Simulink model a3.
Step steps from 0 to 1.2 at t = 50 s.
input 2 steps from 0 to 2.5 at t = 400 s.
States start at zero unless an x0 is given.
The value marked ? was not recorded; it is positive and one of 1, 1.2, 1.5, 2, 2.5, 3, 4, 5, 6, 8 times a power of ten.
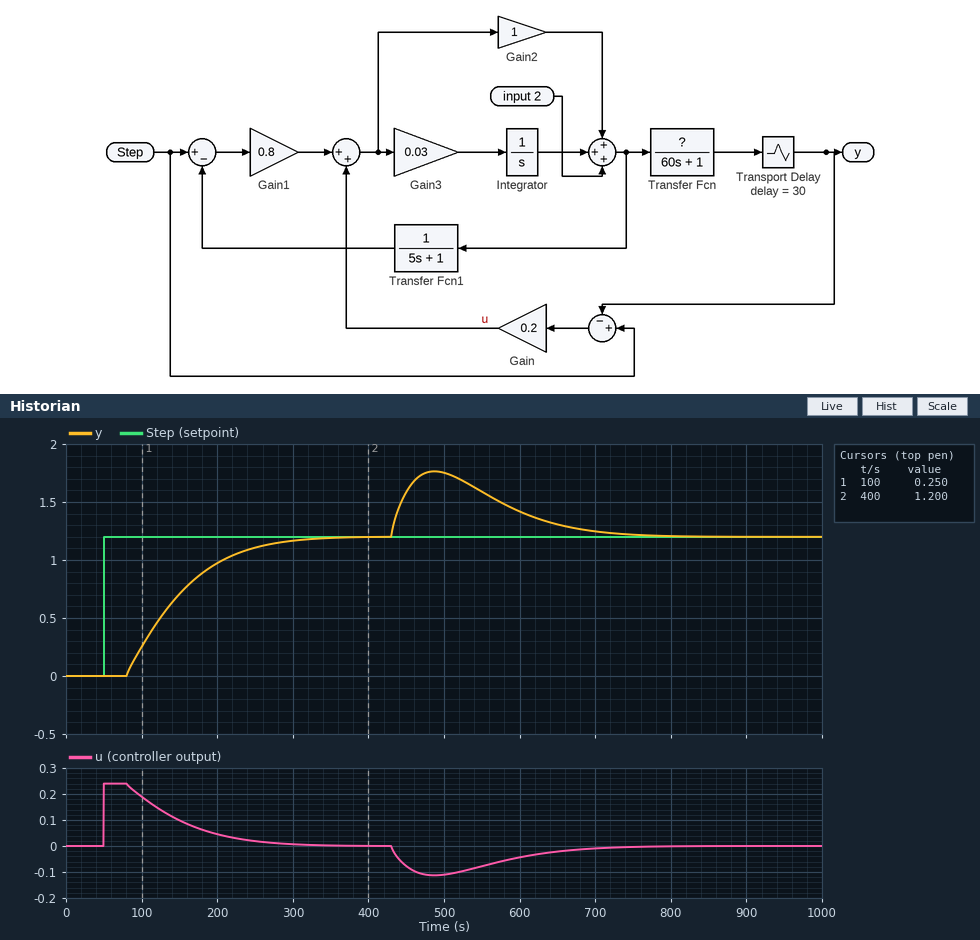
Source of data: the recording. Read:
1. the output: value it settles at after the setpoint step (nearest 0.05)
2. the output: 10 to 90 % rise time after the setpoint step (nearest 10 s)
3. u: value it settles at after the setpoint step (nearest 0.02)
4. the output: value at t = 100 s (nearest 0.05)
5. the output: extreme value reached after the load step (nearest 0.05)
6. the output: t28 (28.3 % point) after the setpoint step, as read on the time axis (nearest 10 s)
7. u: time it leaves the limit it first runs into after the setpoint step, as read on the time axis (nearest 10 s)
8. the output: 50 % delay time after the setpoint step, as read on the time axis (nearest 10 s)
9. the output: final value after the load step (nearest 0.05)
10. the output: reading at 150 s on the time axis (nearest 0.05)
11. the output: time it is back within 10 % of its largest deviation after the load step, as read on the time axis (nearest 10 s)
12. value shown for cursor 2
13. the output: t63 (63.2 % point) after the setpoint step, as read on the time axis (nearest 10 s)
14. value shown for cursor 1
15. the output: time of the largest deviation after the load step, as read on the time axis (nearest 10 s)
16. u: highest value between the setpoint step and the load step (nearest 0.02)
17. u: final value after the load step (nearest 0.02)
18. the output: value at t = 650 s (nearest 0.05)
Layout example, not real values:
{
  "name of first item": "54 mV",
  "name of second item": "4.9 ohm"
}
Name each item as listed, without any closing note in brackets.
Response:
{
  "the output: value it settles at after the setpoint step": "1.20",
  "the output: 10 to 90 % rise time after the setpoint step": "150 s",
  "u: value it settles at after the setpoint step": "0.00",
  "the output: value at t = 100 s": "0.25",
  "the output: extreme value reached after the load step": "1.75",
  "the output: t28 (28.3 % point) after the setpoint step, as read on the time axis": "110 s",
  "u: time it leaves the limit it first runs into after the setpoint step, as read on the time axis": "80 s",
  "the output: 50 % delay time after the setpoint step, as read on the time axis": "140 s",
  "the output: final value after the load step": "1.20",
  "the output: reading at 150 s on the time axis": "0.70",
  "the output: time it is back within 10 % of its largest deviation after the load step, as read on the time axis": "690 s",
  "value shown for cursor 2": "1.200",
  "the output: t63 (63.2 % point) after the setpoint step, as read on the time axis": "160 s",
  "value shown for cursor 1": "0.250",
  "the output: time of the largest deviation after the load step, as read on the time axis": "490 s",
  "u: highest value between the setpoint step and the load step": "0.24",
  "u: final value after the load step": "0.00",
  "the output: value at t = 650 s": "1.30"
}
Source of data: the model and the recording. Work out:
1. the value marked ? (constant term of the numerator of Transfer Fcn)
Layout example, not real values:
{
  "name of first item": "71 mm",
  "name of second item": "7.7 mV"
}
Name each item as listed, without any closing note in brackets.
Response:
{
  "the value marked ?": "1"
}
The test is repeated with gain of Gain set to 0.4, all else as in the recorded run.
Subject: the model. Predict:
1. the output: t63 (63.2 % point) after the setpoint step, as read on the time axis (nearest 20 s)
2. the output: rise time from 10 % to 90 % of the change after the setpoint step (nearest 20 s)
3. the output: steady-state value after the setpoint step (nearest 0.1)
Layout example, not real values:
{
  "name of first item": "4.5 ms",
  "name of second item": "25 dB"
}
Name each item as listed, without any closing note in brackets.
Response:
{
  "the output: t63 (63.2 % point) after the setpoint step, as read on the time axis": "140 s",
  "the output: rise time from 10 % to 90 % of the change after the setpoint step": "120 s",
  "the output: steady-state value after the setpoint step": "1.2"
}
